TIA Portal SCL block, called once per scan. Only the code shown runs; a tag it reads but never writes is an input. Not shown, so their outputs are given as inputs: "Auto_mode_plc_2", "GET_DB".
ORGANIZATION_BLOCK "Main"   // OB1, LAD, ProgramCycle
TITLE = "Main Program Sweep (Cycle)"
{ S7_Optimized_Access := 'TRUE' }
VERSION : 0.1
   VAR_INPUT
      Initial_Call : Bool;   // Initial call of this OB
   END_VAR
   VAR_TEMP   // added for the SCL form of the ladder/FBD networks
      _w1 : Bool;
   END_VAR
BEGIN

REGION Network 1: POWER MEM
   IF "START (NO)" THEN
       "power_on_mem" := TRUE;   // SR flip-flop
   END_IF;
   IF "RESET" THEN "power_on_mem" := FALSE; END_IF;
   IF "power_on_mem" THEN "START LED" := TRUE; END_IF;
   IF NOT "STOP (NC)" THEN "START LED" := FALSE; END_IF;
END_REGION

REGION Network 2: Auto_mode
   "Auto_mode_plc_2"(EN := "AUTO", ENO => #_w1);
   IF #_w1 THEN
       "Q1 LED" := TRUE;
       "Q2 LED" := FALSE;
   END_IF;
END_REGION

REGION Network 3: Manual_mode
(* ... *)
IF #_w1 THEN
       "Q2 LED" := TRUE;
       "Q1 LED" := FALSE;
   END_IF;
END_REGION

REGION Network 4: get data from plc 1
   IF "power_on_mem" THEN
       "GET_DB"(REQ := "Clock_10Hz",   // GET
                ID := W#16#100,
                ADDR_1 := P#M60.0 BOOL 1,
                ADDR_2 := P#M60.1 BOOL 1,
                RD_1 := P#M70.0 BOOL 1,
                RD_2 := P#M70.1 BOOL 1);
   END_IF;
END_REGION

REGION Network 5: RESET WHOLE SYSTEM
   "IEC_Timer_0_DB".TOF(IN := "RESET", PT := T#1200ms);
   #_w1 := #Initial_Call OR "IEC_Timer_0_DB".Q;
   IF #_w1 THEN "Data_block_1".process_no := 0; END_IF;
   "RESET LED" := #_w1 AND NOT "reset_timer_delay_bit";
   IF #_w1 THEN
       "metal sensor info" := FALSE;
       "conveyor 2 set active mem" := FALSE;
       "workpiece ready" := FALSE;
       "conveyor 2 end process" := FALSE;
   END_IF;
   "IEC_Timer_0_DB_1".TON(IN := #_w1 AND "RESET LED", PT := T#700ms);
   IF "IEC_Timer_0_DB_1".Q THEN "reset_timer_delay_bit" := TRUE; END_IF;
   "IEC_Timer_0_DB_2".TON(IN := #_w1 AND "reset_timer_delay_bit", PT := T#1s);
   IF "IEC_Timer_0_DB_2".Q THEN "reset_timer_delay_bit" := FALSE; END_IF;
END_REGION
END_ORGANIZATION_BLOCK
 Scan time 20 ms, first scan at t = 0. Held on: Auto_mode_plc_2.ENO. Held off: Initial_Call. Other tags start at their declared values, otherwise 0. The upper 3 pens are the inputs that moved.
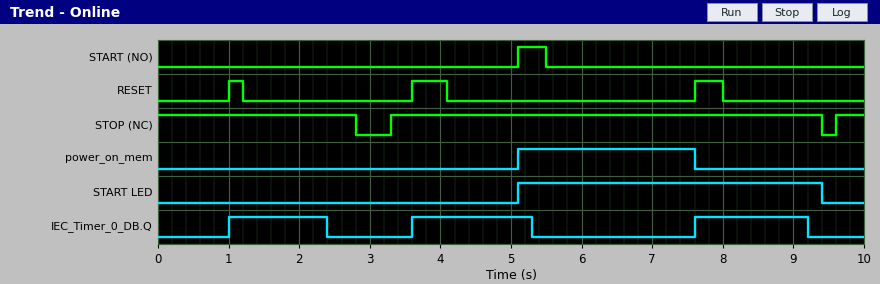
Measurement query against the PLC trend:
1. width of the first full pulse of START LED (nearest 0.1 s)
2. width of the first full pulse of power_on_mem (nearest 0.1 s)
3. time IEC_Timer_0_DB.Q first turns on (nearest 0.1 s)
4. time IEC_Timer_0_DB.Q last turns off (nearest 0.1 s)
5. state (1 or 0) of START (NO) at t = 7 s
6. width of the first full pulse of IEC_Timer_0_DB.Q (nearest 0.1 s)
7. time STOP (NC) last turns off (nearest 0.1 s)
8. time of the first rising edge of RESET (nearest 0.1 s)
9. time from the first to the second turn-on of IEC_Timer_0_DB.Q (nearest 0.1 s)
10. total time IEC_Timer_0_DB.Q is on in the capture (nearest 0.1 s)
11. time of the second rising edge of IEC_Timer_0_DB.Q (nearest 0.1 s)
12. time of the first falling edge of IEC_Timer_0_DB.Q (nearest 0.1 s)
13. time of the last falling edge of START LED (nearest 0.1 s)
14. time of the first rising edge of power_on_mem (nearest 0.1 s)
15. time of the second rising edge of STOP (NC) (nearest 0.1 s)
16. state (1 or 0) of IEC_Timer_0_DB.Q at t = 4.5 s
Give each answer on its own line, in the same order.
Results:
4.3 s
2.5 s
1.0 s
9.2 s
0
1.4 s
9.4 s
1.0 s
2.6 s
4.7 s
3.6 s
2.4 s
9.4 s
5.1 s
9.6 s
1
